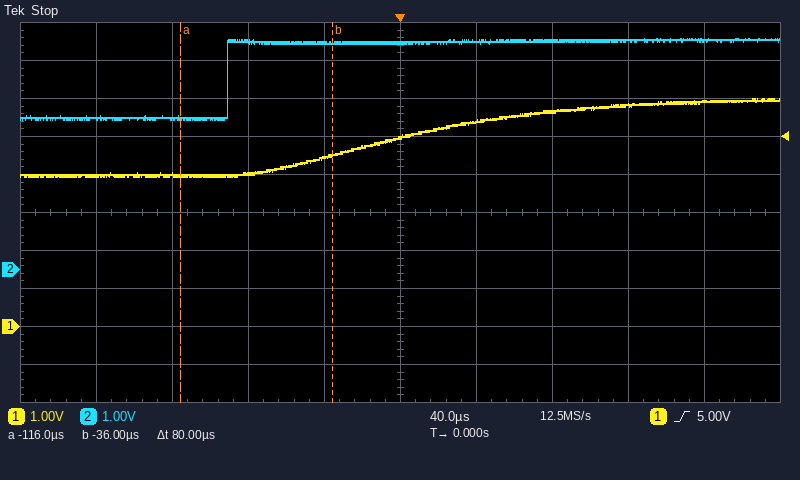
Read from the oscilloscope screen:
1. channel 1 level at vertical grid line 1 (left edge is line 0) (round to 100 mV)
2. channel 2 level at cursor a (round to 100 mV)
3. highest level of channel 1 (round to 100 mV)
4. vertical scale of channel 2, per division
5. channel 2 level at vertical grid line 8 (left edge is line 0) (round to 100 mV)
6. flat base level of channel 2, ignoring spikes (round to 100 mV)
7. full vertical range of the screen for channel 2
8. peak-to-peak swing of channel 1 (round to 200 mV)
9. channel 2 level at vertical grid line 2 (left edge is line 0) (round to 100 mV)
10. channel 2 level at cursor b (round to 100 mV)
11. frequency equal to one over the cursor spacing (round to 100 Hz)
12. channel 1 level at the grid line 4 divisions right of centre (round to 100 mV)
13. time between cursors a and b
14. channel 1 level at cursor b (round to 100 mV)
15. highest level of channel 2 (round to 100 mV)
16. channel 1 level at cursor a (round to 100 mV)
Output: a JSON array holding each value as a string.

["4.0 V", "4.0 V", "6.0 V", "1 V", "6.0 V", "4.0 V", "10 V", "2.0 V", "4.0 V", "6.0 V", "12.5 kHz", "5.9 V", "80 µs", "4.5 V", "6.1 V", "4.0 V"]
